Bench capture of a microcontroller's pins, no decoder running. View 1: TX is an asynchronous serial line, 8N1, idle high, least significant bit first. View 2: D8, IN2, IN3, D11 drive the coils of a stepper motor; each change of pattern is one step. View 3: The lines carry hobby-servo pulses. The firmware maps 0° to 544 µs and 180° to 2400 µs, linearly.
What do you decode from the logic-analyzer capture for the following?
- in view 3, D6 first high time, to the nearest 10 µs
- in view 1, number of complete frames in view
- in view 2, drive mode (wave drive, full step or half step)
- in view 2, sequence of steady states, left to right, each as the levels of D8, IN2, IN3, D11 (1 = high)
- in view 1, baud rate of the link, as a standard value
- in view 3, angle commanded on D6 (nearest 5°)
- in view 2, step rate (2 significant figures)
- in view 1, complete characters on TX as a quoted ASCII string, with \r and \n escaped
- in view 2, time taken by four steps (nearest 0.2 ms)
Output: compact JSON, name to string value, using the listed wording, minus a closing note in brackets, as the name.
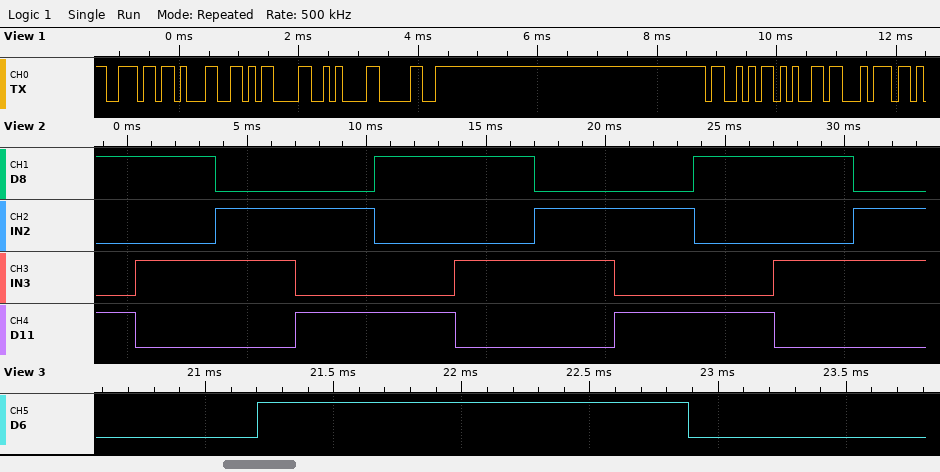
{"in view 3, D6 first high time, to the nearest 10 µs": "1680 µs", "in view 1, number of complete frames in view": "8", "in view 2, drive mode": "full step", "in view 2, sequence of steady states, left to right, each as the levels of D8, IN2, IN3, D11": "1001 1010 0110 0101 1001 1010 0110 0101 1001 1010 0110", "in view 1, baud rate of the link, as a standard value": "9600 baud", "in view 3, angle commanded on D6": "110°", "in view 2, step rate": "300 steps/s", "in view 1, complete characters on TX as a quoted ASCII string, with \\r and \\n escaped": "\"n1\\r\\n0Set\"", "in view 2, time taken by four steps": "13.4 ms"}
